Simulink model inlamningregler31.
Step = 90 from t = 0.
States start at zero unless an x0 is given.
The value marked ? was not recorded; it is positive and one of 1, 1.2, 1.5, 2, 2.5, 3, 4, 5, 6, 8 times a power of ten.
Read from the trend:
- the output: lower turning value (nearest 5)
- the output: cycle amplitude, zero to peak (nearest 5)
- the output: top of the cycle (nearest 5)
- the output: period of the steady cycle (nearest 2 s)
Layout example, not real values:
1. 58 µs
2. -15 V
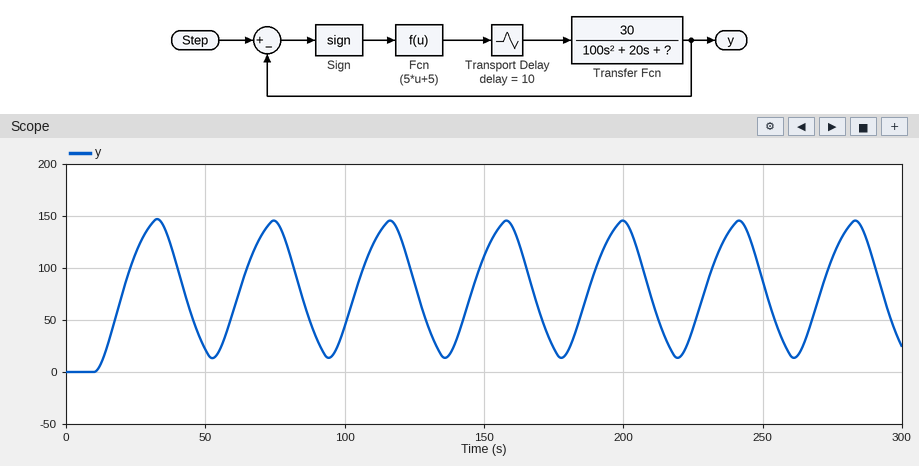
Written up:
1. 15
2. 65
3. 145
4. 42 s
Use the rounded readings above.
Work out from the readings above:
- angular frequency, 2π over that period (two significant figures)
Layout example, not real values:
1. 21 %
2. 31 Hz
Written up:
1. 0.15 rad/s
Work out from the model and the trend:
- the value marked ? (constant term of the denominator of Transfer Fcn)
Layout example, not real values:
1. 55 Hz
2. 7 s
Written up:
1. 2
